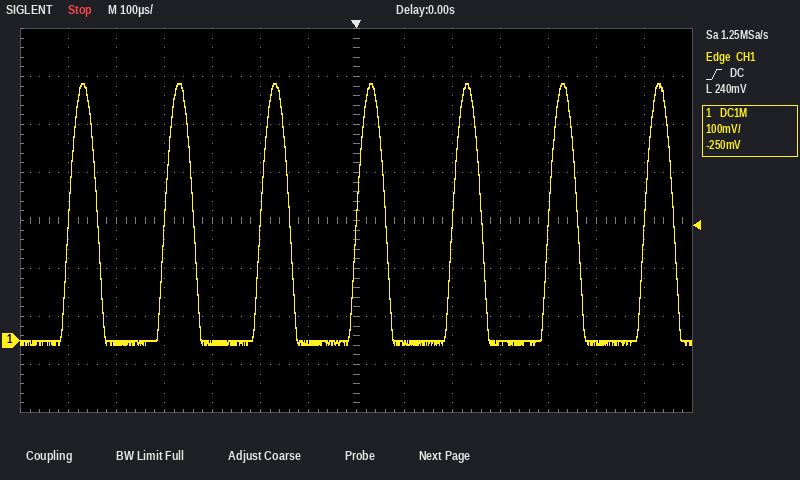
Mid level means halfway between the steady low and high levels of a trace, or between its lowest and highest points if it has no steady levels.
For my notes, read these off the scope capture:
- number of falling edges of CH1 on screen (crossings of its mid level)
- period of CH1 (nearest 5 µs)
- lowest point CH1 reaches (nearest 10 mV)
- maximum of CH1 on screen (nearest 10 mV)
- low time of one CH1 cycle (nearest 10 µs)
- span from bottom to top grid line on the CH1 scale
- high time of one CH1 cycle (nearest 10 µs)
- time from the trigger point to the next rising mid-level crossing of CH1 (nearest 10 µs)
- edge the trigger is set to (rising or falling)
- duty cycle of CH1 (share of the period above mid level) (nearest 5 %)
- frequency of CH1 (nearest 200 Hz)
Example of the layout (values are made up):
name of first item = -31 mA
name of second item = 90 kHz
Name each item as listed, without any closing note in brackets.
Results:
number of falling edges of CH1 on screen = 7
period of CH1 = 200 µs
lowest point CH1 reaches = -10 mV
maximum of CH1 on screen = 540 mV
low time of one CH1 cycle = 140 µs
span from bottom to top grid line on the CH1 scale = 800 mV
high time of one CH1 cycle = 60 µs
time from the trigger point to the next rising mid-level crossing of CH1 = 200 µs
edge the trigger is set to = rising
duty cycle of CH1 (share of the period above mid level) = 30 %
frequency of CH1 = 5.0 kHz
